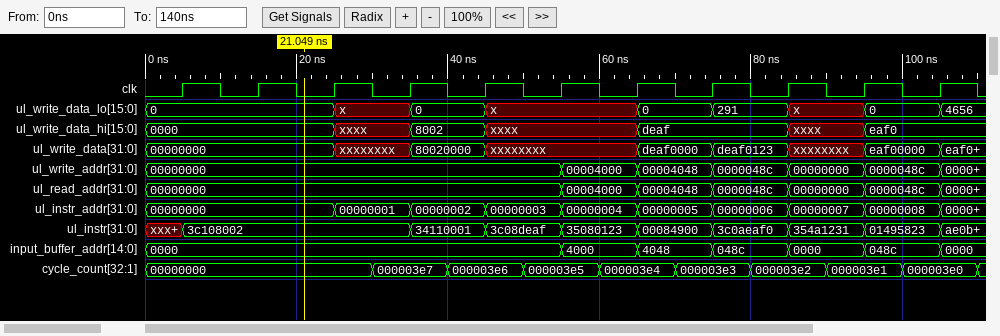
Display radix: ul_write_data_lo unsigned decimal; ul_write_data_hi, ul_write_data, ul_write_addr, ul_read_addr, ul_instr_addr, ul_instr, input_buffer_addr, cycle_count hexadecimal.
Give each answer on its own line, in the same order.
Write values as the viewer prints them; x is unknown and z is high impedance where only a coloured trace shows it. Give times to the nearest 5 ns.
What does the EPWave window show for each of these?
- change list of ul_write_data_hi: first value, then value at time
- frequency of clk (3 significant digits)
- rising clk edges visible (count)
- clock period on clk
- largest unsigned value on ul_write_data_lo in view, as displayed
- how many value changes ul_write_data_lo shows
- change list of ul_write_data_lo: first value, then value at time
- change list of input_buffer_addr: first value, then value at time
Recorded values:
0000, xxxx at 25 ns, 8002 at 35 ns, xxxx at 45 ns, deaf at 65 ns, xxxx at 85 ns, eaf0 at 95 ns
100 MHz
11
10 ns
4656
8
0, x at 25 ns, 0 at 35 ns, x at 45 ns, 0 at 65 ns, 291 at 75 ns, x at 85 ns, 0 at 95 ns, 4656 at 105 ns
0000, 4000 at 55 ns, 4048 at 65 ns, 048c at 75 ns, 0000 at 85 ns, 048c at 95 ns, 0000 at 105 ns
